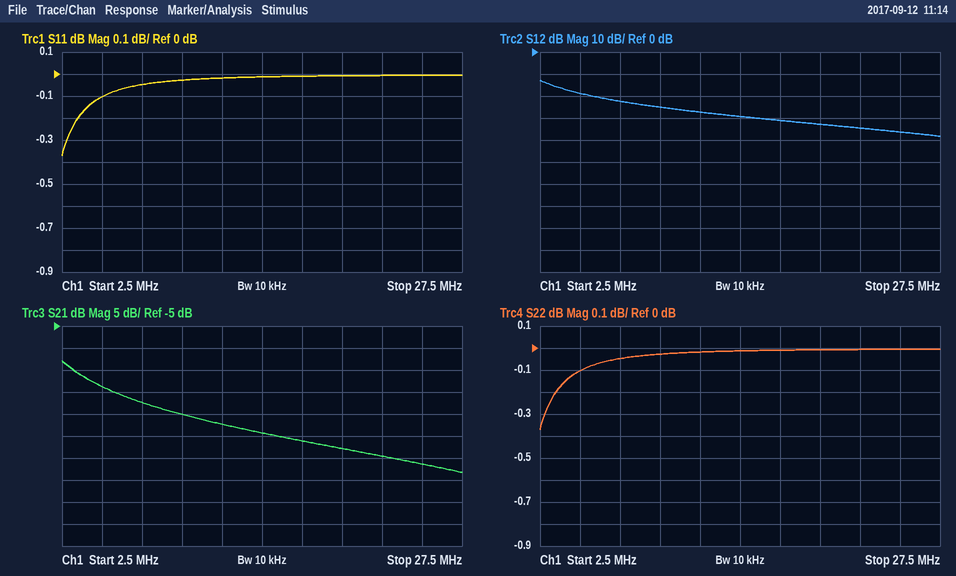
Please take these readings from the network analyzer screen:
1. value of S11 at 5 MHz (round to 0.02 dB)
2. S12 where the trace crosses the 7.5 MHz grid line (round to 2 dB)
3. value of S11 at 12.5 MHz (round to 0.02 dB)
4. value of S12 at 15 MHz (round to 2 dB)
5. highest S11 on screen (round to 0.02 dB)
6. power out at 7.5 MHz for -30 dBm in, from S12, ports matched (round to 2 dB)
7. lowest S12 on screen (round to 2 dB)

-0.10 dB
-22 dB
-0.02 dB
-30 dB
0.00 dB
-52 dBm
-38 dB
